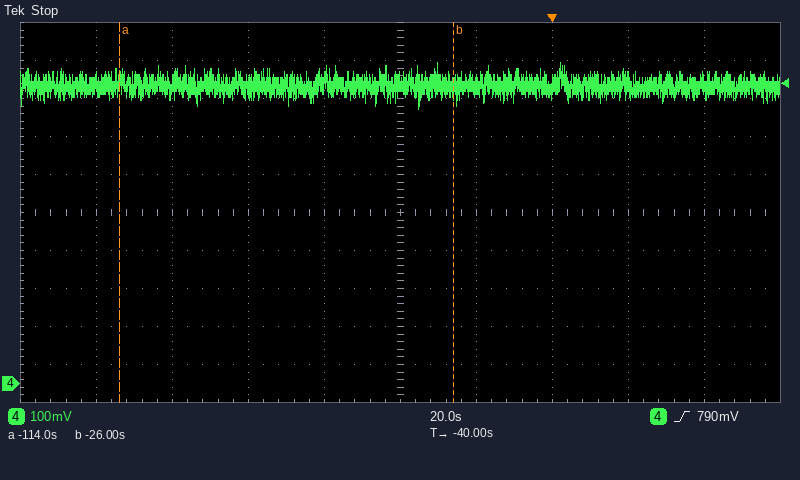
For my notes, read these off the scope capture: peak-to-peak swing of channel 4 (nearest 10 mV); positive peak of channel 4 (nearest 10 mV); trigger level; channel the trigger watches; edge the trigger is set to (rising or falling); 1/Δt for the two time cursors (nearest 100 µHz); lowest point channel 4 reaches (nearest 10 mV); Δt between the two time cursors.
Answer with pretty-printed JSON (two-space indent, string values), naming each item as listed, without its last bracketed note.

{
  "peak-to-peak swing of channel 4": "120 mV",
  "positive peak of channel 4": "840 mV",
  "trigger level": "790 mV",
  "channel the trigger watches": "channel 4",
  "edge the trigger is set to": "rising",
  "1/Δt for the two time cursors": "11.4 mHz",
  "lowest point channel 4 reaches": "720 mV",
  "Δt between the two time cursors": "88 s"
}
